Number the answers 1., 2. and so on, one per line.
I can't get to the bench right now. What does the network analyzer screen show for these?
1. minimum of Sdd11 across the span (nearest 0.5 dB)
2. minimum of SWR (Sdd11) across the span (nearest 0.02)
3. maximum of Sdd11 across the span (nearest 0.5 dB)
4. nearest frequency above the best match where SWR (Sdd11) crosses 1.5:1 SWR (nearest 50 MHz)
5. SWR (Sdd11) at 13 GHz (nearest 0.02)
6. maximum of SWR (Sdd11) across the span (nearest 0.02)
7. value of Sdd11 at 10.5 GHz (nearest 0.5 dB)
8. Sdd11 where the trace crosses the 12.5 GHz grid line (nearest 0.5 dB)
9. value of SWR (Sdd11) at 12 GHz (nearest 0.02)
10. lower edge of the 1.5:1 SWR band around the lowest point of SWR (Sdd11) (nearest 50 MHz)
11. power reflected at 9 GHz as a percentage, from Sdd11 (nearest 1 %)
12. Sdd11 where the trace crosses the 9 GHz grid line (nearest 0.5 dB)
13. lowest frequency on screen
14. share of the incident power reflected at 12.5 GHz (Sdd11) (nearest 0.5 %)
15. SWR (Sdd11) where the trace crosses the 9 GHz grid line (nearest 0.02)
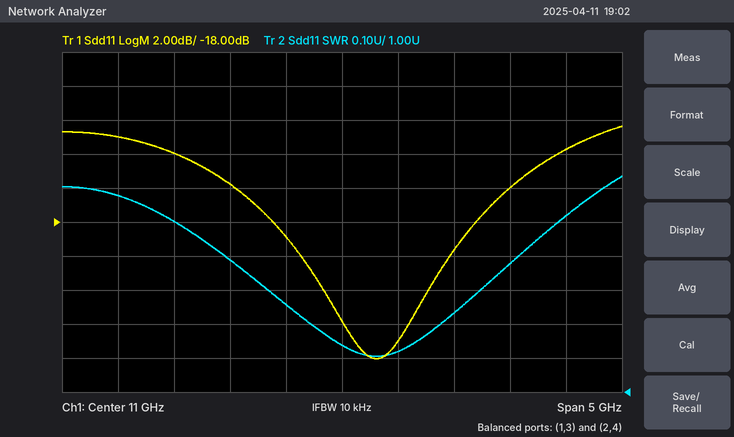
1. -26.0 dB
2. 1.10
3. -12.5 dB
4. 12.95 GHz
5. 1.52
6. 1.64
7. -19.0 dB
8. -16.0 dB
9. 1.24
10. 9.50 GHz
11. 5 %
12. -13.0 dB
13. 8.5 GHz
14. 2.5 %
15. 1.58
